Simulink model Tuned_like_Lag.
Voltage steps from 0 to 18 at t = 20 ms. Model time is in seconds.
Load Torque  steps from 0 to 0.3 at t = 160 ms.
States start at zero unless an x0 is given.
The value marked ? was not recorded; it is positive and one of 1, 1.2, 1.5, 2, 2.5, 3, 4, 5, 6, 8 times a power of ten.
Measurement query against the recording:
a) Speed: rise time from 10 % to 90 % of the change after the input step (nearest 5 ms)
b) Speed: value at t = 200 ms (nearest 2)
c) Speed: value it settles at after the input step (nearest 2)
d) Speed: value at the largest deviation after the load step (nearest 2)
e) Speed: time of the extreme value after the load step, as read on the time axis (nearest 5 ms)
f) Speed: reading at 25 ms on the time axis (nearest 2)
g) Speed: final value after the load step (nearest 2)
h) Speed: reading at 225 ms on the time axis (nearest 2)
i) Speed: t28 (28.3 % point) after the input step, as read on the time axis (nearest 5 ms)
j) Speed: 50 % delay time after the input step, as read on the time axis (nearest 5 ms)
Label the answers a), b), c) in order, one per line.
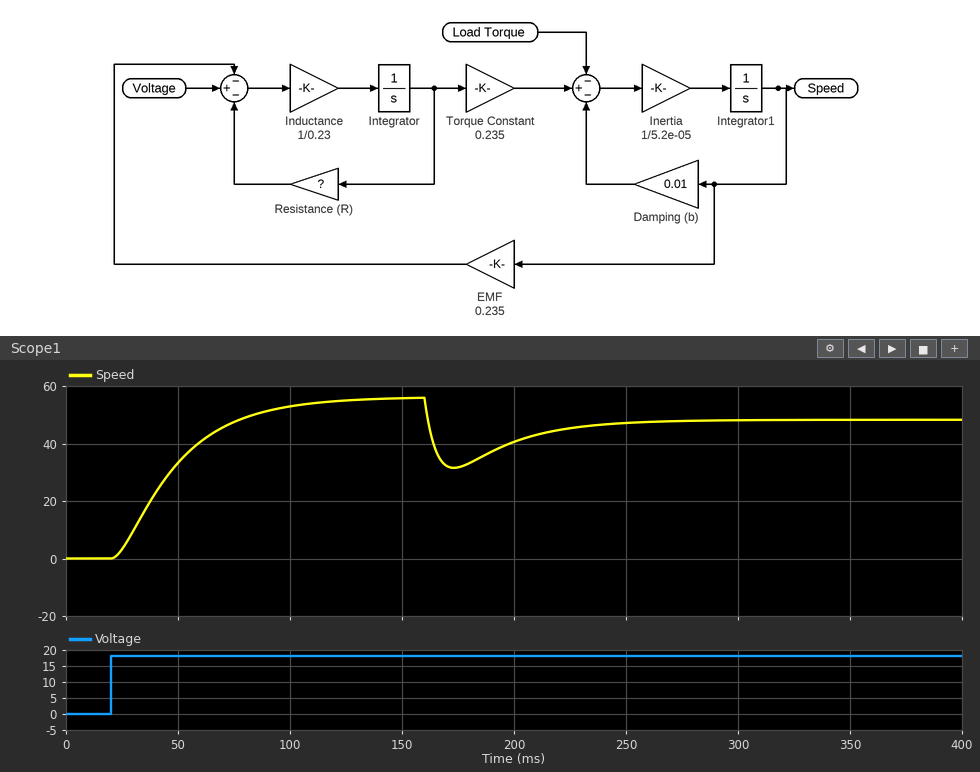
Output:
a) 60 ms
b) 40
c) 56
d) 32
e) 175 ms
f) 4
g) 48
h) 46
i) 35 ms
j) 45 ms
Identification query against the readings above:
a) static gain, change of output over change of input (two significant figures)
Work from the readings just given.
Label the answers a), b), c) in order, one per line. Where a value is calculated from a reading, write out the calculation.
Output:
a) (56 - 0) / (18 - 0) = 3.1
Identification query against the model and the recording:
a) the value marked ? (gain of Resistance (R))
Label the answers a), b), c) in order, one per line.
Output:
a) 2
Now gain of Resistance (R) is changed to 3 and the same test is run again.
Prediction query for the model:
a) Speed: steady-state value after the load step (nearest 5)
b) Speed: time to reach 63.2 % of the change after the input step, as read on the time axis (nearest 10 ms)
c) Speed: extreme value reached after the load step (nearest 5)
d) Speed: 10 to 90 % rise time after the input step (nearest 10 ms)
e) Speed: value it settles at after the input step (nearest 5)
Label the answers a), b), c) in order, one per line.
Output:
a) 40
b) 50 ms
c) 25
d) 50 ms
e) 50
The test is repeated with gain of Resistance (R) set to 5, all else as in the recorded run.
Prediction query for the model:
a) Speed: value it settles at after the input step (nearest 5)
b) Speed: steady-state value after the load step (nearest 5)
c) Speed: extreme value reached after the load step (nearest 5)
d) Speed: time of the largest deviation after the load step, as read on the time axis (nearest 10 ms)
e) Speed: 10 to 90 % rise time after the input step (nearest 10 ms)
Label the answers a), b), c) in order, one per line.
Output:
a) 40
b) 25
c) 15
d) 170 ms
e) 40 ms
